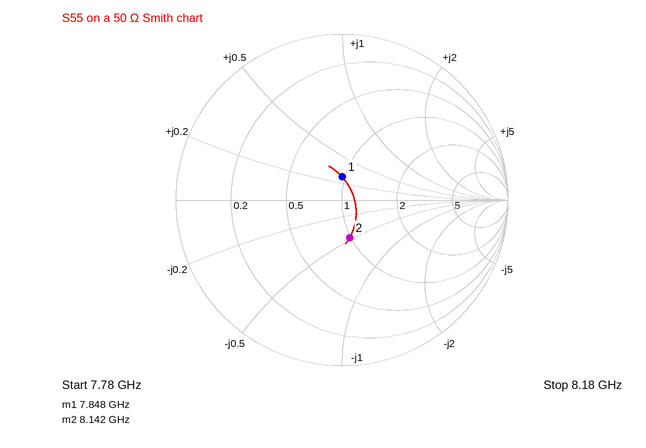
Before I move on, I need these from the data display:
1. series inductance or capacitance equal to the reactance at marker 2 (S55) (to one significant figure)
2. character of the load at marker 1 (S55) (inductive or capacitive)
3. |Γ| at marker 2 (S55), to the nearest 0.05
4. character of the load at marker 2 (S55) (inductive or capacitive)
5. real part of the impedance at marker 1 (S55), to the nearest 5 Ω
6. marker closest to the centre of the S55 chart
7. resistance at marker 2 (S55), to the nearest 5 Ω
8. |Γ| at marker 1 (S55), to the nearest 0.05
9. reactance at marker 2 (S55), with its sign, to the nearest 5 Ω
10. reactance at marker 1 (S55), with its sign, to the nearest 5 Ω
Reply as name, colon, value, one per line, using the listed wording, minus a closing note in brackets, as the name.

series inductance or capacitance equal to the reactance at marker 2 (S55): 800 fF
character of the load at marker 1 (S55): inductive
|Γ| at marker 2 (S55), to the nearest 0.05: 0.25
character of the load at marker 2 (S55): capacitive
real part of the impedance at marker 1 (S55), to the nearest 5 Ω: 50 Ω
marker closest to the centre of the S55 chart: marker 1
resistance at marker 2 (S55), to the nearest 5 Ω: 50 Ω
|Γ| at marker 1 (S55), to the nearest 0.05: 0.15
reactance at marker 2 (S55), with its sign, to the nearest 5 Ω: -25 Ω
reactance at marker 1 (S55), with its sign, to the nearest 5 Ω: +15 Ω
